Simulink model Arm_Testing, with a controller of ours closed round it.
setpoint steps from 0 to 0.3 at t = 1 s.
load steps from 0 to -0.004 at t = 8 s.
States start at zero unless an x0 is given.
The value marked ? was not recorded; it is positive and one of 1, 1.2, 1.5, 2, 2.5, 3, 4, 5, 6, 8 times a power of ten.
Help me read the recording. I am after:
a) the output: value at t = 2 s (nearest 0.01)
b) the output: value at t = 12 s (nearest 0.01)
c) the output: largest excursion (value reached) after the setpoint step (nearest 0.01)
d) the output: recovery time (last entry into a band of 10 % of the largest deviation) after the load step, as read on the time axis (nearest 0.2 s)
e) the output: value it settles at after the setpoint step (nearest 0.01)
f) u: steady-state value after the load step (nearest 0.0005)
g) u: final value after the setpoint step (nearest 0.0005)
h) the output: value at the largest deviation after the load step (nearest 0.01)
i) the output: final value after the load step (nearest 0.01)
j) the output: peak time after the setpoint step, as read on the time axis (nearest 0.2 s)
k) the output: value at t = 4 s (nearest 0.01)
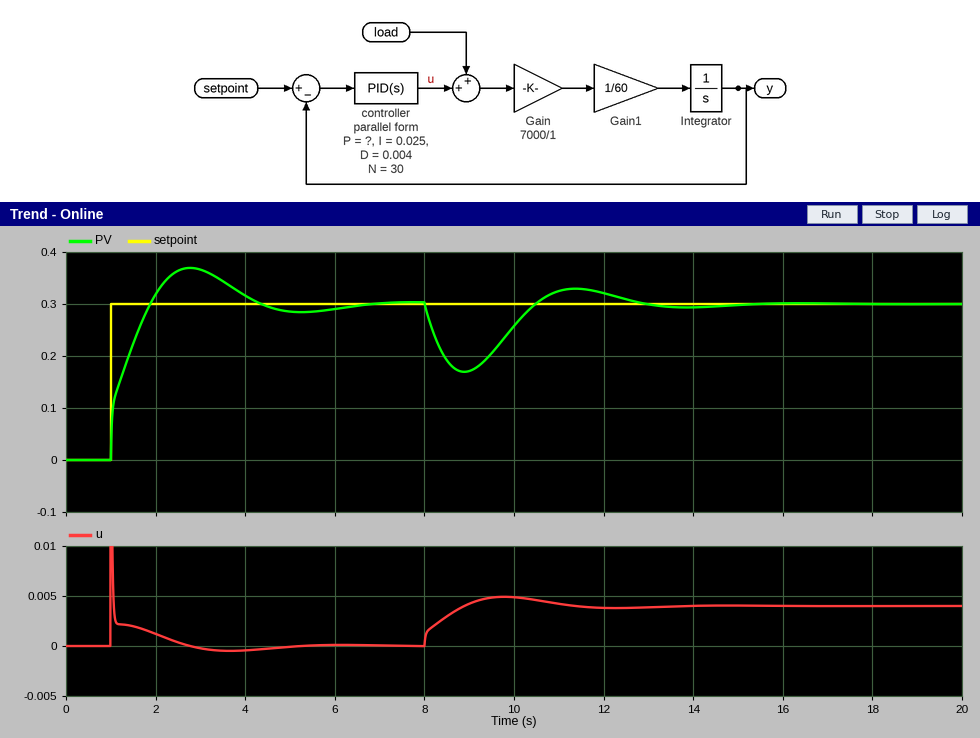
0.32
0.32
0.37
12.4 s
0.30
0.0040
0.0000
0.17
0.30
2.8 s
0.32
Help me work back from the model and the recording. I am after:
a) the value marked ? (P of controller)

0.015
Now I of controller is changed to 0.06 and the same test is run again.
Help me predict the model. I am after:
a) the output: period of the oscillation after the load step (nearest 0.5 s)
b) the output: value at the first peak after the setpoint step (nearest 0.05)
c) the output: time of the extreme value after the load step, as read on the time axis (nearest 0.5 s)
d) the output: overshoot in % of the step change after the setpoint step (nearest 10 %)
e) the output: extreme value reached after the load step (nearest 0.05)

3.0 s
0.40
8.5 s
30 %
0.20
